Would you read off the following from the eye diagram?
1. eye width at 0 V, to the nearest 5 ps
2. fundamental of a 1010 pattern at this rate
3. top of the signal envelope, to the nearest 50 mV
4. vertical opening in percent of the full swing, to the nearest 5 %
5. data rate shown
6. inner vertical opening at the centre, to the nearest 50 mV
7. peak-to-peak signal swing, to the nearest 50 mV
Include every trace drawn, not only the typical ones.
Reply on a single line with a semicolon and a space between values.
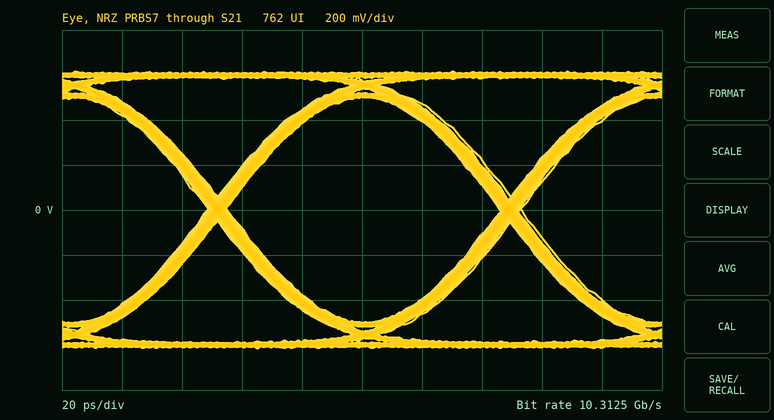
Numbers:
90 ps; 5.15625 GHz; 600 mV; 80 %; 10.3125 Gb/s; 1.00 V; 1.25 V
